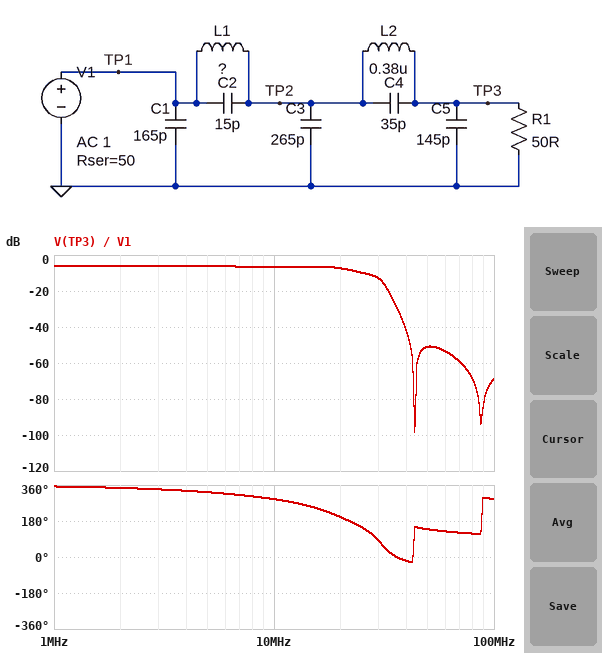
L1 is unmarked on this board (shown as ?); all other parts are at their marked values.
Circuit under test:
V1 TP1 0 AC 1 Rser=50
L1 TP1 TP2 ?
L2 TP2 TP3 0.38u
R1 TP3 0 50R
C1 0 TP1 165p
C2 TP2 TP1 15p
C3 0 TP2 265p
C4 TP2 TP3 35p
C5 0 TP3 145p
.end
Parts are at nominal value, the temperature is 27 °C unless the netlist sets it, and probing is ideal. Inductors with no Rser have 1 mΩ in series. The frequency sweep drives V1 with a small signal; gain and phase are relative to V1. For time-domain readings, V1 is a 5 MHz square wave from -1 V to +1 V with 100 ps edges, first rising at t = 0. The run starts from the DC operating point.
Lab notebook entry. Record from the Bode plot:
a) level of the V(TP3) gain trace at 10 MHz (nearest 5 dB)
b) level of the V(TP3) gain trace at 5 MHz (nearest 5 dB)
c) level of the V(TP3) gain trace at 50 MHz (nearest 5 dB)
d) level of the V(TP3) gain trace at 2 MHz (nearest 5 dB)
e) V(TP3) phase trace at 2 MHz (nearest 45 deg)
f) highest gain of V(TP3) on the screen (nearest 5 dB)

-5 dB
-5 dB
-50 dB
-5 dB
360 deg
-5 dB
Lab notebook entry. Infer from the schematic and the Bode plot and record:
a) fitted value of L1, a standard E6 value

220 nH
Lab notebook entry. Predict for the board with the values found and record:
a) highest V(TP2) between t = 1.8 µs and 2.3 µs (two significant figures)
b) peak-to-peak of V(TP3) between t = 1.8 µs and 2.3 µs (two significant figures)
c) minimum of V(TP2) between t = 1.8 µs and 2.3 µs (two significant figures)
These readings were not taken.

620 mV
1.2 V
-620 mV
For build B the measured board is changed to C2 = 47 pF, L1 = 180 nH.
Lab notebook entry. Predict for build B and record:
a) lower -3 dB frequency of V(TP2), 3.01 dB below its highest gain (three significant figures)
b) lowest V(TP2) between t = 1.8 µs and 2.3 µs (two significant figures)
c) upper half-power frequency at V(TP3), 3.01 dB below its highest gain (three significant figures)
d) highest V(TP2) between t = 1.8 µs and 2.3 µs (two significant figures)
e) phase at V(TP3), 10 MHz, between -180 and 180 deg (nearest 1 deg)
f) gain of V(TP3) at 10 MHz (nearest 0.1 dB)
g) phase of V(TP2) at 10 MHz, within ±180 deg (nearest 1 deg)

24.2 MHz
-600 mV
22.9 MHz
600 mV
-69 deg
-6.6 dB
-36 deg
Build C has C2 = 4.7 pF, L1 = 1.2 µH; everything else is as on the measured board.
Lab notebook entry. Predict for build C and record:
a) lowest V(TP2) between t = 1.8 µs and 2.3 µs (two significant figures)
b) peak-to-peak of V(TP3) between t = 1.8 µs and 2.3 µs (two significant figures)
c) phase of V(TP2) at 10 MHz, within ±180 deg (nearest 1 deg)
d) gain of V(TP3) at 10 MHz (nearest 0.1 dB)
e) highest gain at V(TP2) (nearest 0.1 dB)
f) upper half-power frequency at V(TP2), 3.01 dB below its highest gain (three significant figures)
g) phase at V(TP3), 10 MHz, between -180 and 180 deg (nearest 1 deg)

-530 mV
1.1 V
-85 deg
-7.2 dB
-6.0 dB
12.0 MHz
-118 deg
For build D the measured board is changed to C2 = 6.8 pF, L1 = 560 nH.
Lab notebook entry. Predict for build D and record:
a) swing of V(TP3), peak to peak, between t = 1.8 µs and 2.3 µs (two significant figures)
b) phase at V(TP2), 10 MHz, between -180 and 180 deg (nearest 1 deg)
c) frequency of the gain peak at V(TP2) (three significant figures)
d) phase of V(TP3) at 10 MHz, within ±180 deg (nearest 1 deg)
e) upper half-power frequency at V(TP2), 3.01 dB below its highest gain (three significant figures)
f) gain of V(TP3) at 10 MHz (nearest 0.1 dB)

1.3 V
-54 deg
22.3 MHz
-87 deg
25.0 MHz
-6.1 dB
